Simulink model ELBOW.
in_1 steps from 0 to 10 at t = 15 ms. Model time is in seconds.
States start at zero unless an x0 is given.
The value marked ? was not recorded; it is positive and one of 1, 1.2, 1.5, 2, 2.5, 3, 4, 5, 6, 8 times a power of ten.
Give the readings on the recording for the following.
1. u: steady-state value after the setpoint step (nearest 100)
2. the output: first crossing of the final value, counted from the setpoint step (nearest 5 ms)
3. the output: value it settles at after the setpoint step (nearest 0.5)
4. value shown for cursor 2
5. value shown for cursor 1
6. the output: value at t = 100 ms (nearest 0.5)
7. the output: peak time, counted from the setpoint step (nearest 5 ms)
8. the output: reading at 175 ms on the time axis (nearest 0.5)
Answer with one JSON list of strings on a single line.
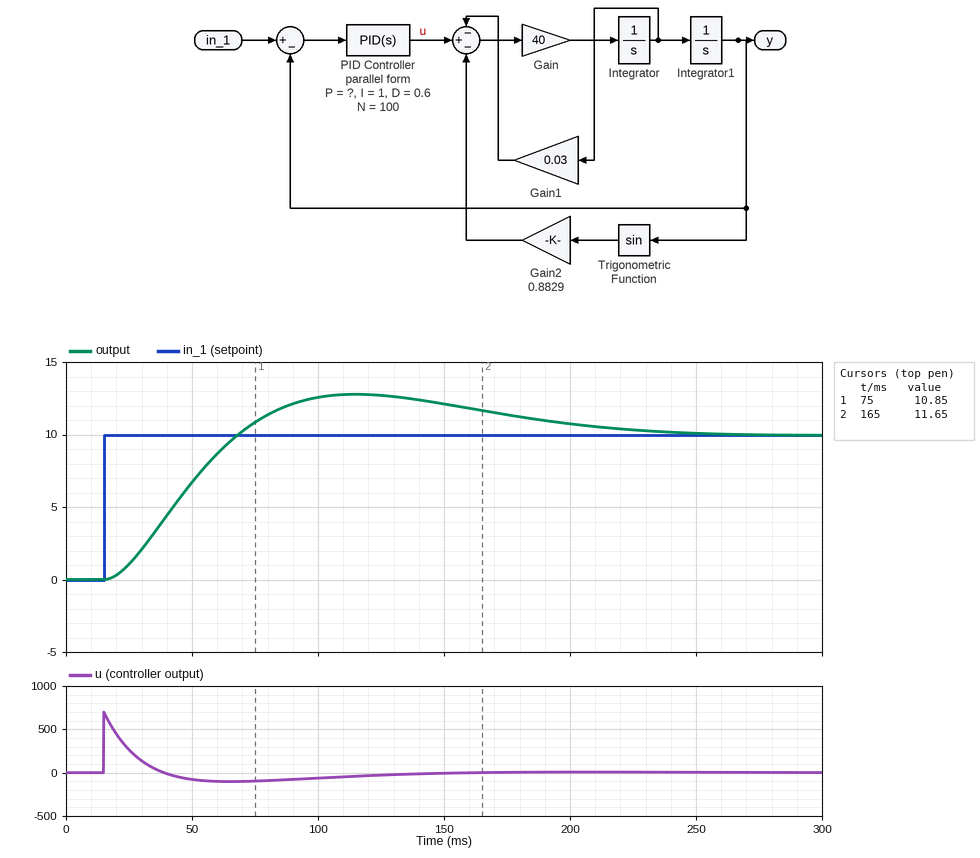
["0", "55 ms", "10.0", "11.65", "10.85", "12.5", "100 ms", "11.5"]
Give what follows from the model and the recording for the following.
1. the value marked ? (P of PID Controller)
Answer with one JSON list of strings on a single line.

["10"]
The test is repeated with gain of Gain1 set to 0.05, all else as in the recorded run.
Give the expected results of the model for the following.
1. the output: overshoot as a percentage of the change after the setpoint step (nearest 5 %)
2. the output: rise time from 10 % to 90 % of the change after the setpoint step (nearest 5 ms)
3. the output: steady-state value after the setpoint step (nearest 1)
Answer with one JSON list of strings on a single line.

["25 %", "40 ms", "10"]
